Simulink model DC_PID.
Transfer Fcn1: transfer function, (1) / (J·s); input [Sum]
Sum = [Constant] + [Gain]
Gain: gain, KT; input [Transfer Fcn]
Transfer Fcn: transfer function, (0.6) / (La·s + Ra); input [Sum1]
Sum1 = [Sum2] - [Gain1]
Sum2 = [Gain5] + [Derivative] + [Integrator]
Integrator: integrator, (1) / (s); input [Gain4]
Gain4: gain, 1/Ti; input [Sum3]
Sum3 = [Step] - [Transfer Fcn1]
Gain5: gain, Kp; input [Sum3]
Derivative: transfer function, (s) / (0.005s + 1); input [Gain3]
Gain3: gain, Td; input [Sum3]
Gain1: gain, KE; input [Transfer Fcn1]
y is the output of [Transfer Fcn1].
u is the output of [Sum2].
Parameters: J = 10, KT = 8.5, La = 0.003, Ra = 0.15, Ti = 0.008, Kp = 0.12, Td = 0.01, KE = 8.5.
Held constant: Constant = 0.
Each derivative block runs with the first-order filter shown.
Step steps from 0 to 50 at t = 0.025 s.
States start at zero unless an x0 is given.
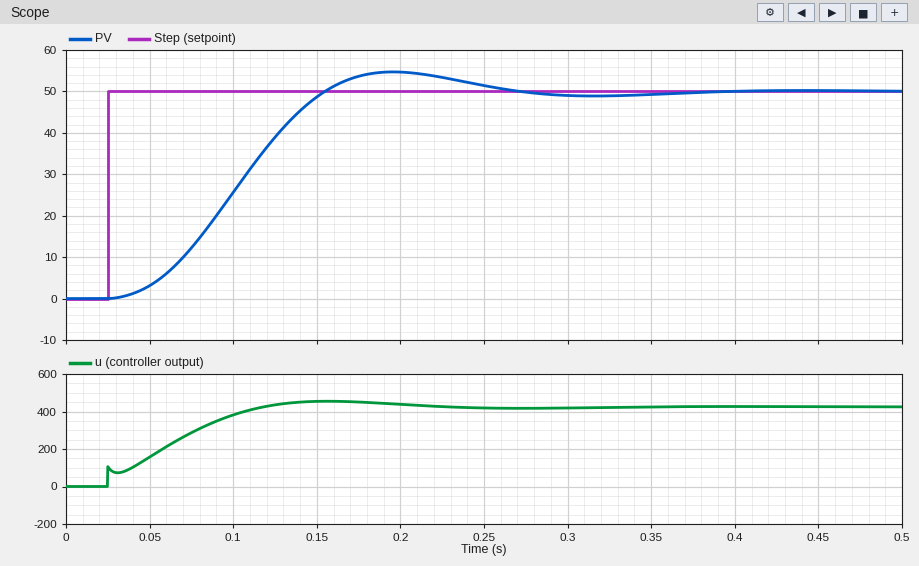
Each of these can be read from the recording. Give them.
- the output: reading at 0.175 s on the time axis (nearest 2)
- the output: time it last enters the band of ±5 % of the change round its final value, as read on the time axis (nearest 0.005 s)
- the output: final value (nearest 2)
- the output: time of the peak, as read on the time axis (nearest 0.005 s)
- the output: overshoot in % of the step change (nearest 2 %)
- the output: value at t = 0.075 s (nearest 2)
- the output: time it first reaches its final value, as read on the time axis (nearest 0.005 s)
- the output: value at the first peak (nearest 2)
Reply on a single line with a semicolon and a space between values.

54; 0.235 s; 50; 0.195 s; 10 %; 12; 0.155 s; 54
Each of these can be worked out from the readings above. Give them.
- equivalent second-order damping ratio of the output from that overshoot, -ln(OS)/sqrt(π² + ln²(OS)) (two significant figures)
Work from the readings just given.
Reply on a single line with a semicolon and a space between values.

0.59
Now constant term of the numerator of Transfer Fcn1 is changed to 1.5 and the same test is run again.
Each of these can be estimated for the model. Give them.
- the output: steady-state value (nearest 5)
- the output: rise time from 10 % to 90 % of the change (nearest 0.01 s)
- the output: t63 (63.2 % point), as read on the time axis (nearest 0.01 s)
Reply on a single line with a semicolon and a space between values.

50; 0.08 s; 0.10 s
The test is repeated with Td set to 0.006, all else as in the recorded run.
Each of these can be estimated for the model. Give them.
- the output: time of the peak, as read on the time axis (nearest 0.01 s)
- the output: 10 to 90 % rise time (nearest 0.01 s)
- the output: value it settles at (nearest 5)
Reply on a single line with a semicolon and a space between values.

0.19 s; 0.08 s; 50
